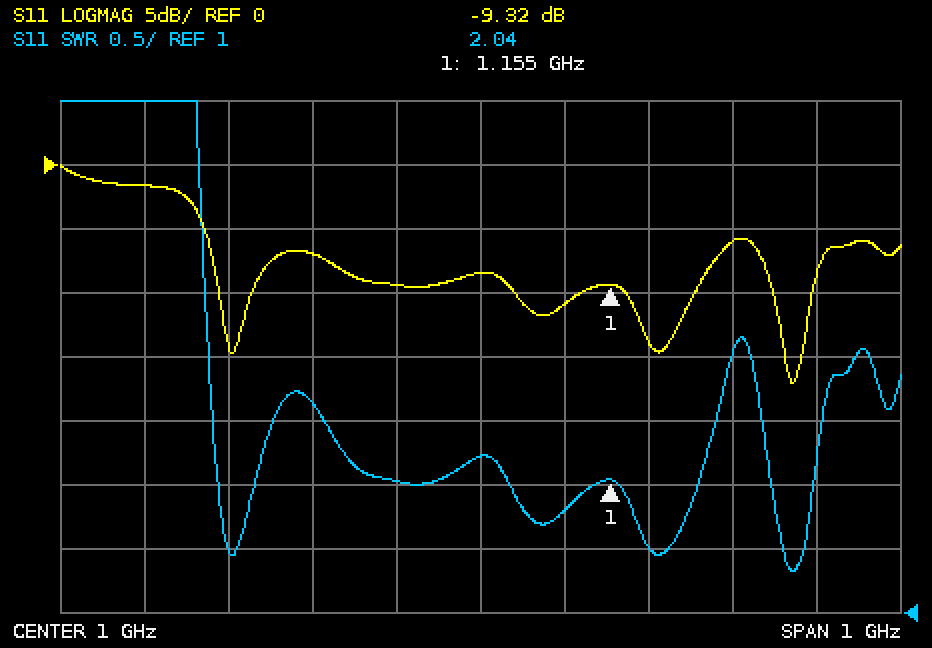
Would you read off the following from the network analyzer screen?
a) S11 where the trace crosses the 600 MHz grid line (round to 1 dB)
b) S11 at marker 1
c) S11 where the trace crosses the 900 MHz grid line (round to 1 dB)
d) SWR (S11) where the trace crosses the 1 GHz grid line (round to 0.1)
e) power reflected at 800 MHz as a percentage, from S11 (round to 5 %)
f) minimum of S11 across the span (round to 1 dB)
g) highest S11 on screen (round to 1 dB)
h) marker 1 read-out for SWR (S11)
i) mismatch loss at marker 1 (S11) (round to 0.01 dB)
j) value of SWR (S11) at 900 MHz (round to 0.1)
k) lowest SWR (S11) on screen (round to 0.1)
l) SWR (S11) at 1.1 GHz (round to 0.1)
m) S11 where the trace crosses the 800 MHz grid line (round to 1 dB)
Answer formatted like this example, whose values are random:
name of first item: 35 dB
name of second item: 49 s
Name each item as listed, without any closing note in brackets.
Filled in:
S11 where the trace crosses the 600 MHz grid line: -2 dB
S11 at marker 1: -9.32 dB
S11 where the trace crosses the 900 MHz grid line: -9 dB
SWR (S11) where the trace crosses the 1 GHz grid line: 2.2
power reflected at 800 MHz as a percentage, from S11: 20 %
minimum of S11 across the span: -17 dB
highest S11 on screen: 0 dB
marker 1 read-out for SWR: 2.04
mismatch loss at marker 1 (S11): 0.54 dB
value of SWR (S11) at 900 MHz: 2.0
lowest SWR (S11) on screen: 1.3
SWR (S11) at 1.1 GHz: 1.8
S11 where the trace crosses the 800 MHz grid line: -7 dB
